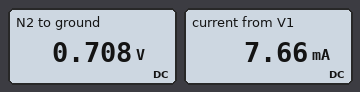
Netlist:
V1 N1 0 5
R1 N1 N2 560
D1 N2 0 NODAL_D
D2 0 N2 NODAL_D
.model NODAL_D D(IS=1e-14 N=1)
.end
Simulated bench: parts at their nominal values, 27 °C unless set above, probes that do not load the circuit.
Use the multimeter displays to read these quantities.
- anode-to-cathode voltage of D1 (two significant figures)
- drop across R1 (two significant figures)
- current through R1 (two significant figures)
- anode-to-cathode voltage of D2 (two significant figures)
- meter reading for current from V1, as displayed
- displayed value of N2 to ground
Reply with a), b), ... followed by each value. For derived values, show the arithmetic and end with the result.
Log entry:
a) 708 mV = 710 mV
b) 5 V - 708 mV = 4.3 V
c) (5 V - 708 mV) / 560 Ω = 7.7 mA
d) 0 V - 708 mV = -710 mV
e) 7.66 mA
f) 0.708 V
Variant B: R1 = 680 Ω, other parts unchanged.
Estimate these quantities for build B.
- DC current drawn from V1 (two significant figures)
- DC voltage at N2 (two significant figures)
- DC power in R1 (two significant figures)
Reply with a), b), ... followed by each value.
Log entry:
a) 6.3 mA
b) 700 mV
c) 27 mW
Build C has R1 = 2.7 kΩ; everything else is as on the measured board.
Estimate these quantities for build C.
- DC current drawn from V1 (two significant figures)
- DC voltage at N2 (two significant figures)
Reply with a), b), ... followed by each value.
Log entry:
a) 1.6 mA
b) 670 mV
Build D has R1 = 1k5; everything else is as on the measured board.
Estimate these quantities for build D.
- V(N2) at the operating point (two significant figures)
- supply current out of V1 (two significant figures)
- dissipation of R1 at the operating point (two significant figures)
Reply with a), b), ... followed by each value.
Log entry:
a) 680 mV
b) 2.9 mA
c) 12 mW
